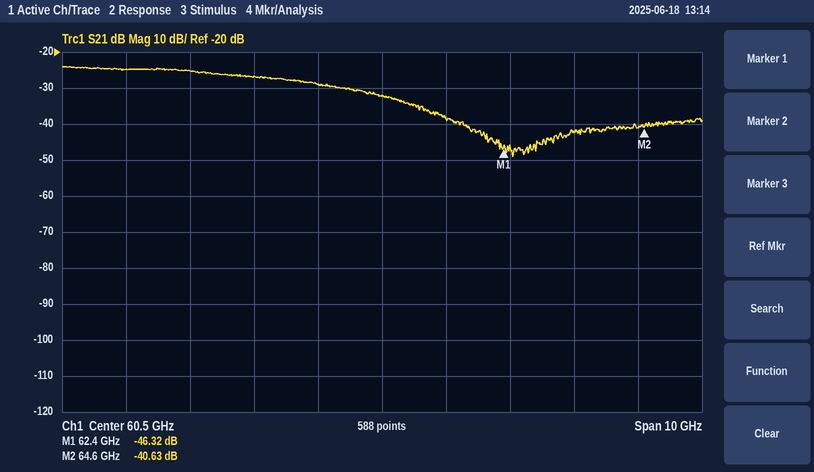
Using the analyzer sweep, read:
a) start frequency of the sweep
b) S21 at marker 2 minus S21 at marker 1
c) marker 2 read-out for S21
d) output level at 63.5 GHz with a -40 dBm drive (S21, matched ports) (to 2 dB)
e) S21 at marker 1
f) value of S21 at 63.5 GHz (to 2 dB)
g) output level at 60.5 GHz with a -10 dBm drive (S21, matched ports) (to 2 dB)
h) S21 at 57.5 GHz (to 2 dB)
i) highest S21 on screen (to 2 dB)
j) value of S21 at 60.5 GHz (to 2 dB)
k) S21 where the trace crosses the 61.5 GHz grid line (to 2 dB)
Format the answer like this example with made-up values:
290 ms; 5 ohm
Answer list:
55.5 GHz; 5.69 dB; -40.63 dB; -82 dBm; -46.32 dB; -42 dB; -42 dBm; -26 dB; -24 dB; -32 dB; -38 dB
